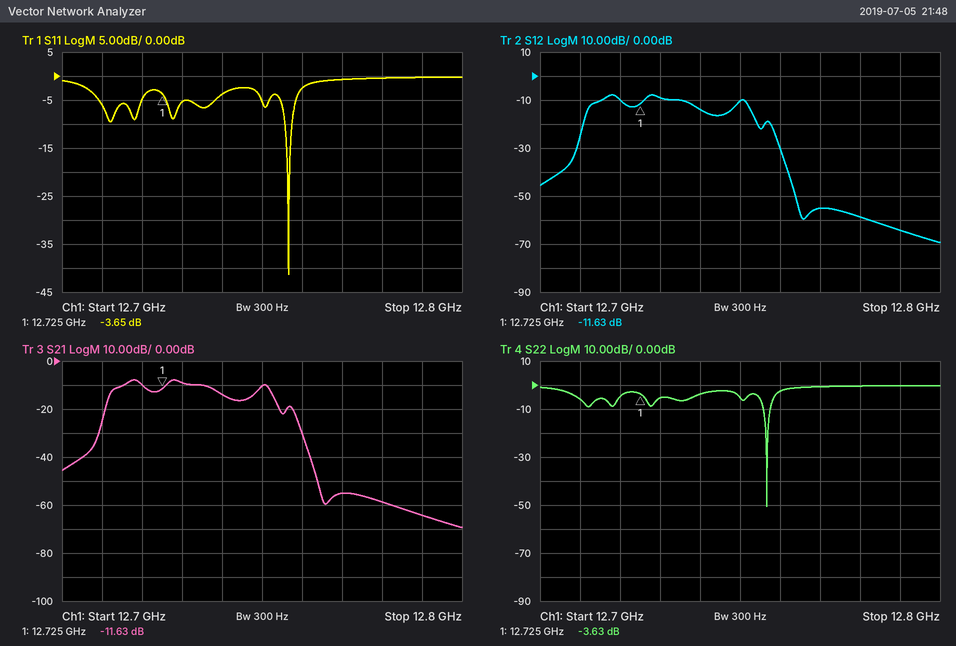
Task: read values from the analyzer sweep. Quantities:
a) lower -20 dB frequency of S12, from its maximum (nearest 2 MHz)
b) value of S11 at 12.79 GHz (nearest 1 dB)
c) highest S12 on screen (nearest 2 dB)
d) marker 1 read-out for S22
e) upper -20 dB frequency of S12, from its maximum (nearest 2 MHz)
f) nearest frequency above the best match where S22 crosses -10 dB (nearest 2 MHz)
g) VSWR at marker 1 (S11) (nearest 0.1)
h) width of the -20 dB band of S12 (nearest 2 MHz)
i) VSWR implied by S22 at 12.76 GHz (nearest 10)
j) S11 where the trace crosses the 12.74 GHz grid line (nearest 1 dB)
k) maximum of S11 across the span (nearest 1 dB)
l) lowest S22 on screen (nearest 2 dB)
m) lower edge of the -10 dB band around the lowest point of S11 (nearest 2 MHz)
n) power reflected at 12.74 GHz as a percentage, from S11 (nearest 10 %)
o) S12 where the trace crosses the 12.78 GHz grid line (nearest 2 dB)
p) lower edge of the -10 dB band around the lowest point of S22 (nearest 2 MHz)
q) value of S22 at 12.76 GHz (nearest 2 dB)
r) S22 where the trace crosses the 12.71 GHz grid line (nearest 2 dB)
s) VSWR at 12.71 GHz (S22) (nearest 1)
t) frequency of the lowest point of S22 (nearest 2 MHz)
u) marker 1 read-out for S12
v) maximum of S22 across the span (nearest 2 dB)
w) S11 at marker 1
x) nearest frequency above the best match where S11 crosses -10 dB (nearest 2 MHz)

12.710 GHz
0 dB
-8 dB
-3.63 dB
12.760 GHz
12.758 GHz
4.8
50 MHz
10
-4 dB
0 dB
-50 dB
12.756 GHz
40 %
-58 dB
12.756 GHz
-2 dB
-6 dB
3
12.756 GHz
-11.63 dB
0 dB
-3.65 dB
12.758 GHz
